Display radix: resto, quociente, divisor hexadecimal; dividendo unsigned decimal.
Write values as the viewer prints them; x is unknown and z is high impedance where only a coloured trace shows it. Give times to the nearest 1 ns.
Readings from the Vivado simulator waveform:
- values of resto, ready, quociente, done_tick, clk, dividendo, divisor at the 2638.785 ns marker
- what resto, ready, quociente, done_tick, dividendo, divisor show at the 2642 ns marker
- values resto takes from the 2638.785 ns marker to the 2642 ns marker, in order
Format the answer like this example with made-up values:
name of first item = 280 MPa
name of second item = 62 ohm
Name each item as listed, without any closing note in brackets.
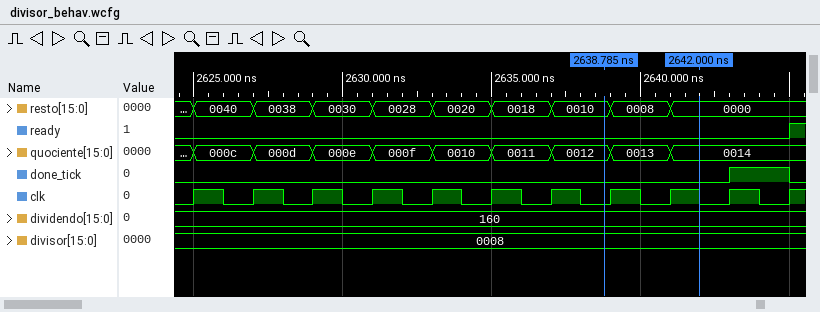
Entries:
values of resto, ready, quociente, done_tick, clk, dividendo, divisor at the 2638.785 ns marker = resto=0010, ready=0, quociente=0012, done_tick=0, clk=0, dividendo=160, divisor=0008
what resto, ready, quociente, done_tick, dividendo, divisor show at the 2642 ns marker = resto=0000, ready=0, quociente=0014, done_tick=0, dividendo=160, divisor=0008
values resto takes from the 2638.785 ns marker to the 2642 ns marker, in order = 0010, 0008, 0000
